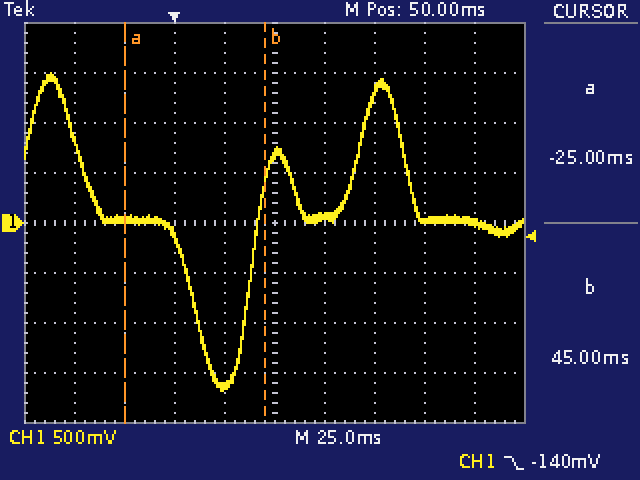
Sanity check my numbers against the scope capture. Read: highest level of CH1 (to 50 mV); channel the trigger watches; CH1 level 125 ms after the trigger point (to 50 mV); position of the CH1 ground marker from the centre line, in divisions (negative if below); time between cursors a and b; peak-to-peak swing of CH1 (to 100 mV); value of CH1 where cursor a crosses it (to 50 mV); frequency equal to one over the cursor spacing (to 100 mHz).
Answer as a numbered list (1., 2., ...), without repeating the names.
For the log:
1. 1.50 V
2. CH1
3. 0 mV
4. 0.0 div
5. 70.0 ms
6. 3.20 V
7. 50 mV
8. 14.3 Hz
